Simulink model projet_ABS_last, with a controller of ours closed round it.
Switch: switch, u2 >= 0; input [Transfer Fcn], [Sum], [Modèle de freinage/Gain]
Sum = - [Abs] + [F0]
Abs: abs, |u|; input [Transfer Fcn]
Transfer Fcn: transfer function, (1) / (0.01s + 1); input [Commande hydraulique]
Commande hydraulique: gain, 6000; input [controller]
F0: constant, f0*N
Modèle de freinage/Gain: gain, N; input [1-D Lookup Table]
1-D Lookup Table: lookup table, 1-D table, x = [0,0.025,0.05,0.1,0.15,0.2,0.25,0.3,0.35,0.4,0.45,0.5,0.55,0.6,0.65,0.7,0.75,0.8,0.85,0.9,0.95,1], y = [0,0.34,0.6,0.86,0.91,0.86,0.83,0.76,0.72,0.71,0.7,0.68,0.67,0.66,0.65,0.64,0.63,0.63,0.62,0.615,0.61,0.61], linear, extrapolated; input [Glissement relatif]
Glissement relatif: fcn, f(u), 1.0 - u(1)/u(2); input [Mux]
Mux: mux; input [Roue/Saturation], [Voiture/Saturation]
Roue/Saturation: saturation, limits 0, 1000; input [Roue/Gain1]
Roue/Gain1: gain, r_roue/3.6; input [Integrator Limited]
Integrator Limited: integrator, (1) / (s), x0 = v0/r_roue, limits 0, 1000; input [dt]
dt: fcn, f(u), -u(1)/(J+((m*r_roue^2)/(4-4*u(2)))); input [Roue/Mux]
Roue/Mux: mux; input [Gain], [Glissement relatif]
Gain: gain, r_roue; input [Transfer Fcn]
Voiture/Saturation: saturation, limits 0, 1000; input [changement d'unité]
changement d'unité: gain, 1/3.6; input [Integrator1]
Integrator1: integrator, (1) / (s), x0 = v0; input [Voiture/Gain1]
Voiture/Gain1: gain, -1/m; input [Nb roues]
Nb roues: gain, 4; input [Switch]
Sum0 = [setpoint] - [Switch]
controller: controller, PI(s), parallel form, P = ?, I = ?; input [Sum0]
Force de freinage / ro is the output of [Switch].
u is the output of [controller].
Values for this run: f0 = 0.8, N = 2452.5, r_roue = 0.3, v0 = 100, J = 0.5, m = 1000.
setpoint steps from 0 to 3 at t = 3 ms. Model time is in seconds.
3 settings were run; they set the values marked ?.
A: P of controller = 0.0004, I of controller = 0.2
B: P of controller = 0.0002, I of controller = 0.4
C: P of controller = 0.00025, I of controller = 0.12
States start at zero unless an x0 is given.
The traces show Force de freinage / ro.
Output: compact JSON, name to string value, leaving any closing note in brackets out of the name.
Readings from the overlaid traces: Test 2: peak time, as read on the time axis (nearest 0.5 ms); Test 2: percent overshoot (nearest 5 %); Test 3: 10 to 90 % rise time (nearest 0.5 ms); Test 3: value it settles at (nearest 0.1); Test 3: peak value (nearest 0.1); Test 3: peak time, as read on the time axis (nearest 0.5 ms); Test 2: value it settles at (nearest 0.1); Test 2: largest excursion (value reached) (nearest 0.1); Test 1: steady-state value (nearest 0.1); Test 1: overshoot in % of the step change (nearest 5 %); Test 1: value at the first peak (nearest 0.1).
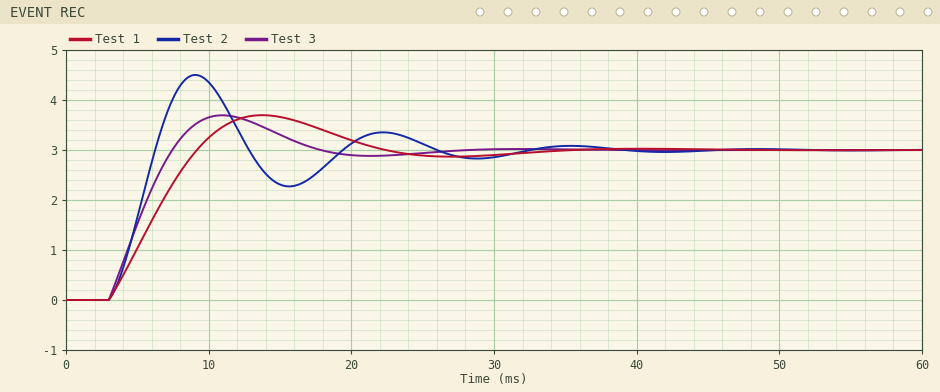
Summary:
{"Test 2: peak time, as read on the time axis": "9.0 ms", "Test 2: percent overshoot": "50 %", "Test 3: 10 to 90 % rise time": "3.5 ms", "Test 3: value it settles at": "3.0", "Test 3: peak value": "3.7", "Test 3: peak time, as read on the time axis": "11.0 ms", "Test 2: value it settles at": "3.0", "Test 2: largest excursion (value reached)": "4.5", "Test 1: steady-state value": "3.0", "Test 1: overshoot in % of the step change": "25 %", "Test 1: value at the first peak": "3.7"}
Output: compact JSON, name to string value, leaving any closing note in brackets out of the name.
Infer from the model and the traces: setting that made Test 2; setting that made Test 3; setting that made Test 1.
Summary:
{"setting that made Test 2": "B", "setting that made Test 3": "A", "setting that made Test 1": "C"}
